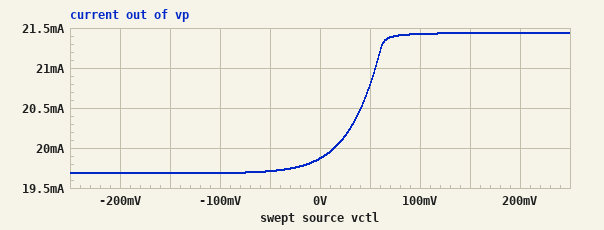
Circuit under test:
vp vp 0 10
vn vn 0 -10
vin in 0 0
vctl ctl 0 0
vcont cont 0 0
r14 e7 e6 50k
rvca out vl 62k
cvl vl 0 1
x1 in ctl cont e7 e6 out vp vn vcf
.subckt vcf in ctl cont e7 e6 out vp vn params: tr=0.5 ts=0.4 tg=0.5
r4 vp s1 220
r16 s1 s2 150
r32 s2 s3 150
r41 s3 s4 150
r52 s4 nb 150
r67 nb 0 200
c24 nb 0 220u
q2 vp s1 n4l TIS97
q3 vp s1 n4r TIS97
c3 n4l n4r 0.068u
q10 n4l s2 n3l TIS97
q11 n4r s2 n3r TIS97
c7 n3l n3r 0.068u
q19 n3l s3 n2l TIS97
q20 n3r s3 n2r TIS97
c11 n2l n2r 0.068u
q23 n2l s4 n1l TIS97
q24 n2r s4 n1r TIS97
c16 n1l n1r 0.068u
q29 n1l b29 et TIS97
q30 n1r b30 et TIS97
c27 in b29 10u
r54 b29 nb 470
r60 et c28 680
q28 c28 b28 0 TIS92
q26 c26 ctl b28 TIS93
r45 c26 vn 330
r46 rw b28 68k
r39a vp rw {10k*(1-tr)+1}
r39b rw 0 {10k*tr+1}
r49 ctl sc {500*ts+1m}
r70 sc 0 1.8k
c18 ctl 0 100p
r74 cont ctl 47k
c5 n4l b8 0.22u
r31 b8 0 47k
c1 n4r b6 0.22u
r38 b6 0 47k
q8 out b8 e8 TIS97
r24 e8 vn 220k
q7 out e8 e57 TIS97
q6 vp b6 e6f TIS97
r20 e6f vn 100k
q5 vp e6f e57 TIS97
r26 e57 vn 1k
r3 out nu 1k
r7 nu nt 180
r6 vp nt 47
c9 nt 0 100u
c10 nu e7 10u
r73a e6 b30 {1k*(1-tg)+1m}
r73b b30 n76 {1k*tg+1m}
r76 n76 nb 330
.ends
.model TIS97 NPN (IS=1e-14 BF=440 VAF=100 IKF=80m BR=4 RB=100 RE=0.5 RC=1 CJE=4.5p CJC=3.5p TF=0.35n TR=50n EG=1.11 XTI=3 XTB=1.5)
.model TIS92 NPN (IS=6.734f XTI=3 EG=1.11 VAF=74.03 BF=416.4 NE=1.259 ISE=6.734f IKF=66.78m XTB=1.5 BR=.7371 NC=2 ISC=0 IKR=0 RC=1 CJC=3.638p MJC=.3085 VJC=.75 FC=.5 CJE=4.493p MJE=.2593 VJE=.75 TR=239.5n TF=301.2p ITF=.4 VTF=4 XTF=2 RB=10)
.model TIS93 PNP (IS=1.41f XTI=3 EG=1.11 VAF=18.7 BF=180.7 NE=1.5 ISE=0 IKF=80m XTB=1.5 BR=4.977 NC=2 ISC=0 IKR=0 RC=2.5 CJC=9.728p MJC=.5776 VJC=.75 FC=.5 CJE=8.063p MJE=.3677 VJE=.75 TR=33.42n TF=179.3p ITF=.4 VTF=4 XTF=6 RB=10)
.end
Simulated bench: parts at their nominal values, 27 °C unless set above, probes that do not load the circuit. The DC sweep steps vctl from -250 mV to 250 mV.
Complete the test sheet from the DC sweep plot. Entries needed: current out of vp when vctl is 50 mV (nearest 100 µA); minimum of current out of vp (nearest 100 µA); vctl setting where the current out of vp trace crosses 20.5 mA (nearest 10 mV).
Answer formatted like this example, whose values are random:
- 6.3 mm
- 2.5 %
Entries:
- 20.8 mA
- 19.7 mA
- 40 mV
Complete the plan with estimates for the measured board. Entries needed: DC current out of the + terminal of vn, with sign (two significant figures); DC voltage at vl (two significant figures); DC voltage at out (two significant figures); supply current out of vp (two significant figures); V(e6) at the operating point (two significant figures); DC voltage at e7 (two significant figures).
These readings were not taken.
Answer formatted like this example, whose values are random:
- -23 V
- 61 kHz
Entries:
- -8.9 mA
- 3.2 V
- 3.2 V
- 20 mA
- 2.0 V
- 2.0 V
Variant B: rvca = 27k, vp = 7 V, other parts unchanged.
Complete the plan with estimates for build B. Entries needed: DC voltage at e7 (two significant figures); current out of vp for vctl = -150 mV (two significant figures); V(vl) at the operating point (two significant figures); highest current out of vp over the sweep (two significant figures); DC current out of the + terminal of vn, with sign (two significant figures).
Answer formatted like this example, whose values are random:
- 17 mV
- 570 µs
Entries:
- 1.4 V
- 16 mA
- 230 mV
- 17 mA
- -8.9 mA
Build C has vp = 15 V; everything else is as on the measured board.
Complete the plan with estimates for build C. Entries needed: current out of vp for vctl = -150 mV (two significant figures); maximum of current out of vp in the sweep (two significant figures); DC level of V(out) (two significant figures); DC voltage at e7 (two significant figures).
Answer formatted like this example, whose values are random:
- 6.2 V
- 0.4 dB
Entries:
- 25 mA
- 28 mA
- 8.2 V
- 2.9 V
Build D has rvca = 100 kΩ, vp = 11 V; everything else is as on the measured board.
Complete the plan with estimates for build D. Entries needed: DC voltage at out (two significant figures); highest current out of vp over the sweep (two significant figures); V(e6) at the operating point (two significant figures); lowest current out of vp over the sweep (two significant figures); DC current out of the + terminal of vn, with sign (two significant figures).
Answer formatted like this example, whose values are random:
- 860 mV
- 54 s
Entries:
- 4.2 V
- 23 mA
- 2.2 V
- 21 mA
- -8.9 mA
